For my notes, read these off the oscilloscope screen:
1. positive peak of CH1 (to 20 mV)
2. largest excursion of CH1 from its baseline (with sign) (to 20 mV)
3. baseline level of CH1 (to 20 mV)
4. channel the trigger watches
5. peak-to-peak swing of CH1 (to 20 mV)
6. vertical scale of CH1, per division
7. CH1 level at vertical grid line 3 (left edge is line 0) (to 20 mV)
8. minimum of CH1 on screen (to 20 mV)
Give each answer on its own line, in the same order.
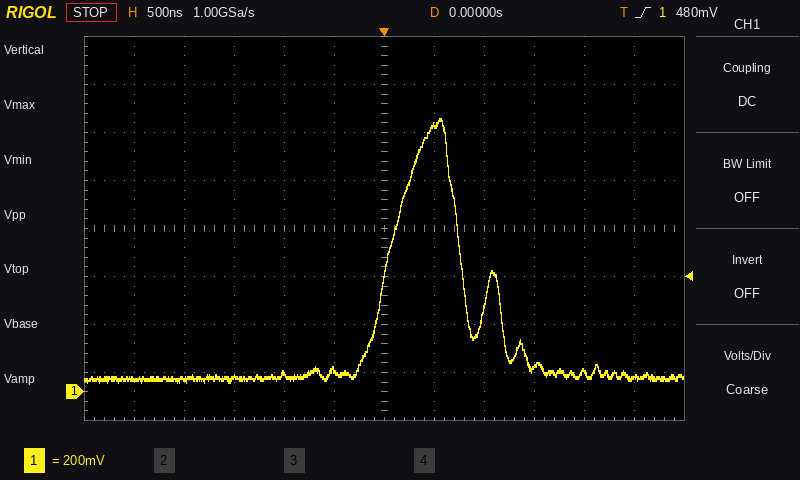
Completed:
1.14 V
+1.08 V
60 mV
CH1
1.10 V
200 mV
60 mV
40 mV
